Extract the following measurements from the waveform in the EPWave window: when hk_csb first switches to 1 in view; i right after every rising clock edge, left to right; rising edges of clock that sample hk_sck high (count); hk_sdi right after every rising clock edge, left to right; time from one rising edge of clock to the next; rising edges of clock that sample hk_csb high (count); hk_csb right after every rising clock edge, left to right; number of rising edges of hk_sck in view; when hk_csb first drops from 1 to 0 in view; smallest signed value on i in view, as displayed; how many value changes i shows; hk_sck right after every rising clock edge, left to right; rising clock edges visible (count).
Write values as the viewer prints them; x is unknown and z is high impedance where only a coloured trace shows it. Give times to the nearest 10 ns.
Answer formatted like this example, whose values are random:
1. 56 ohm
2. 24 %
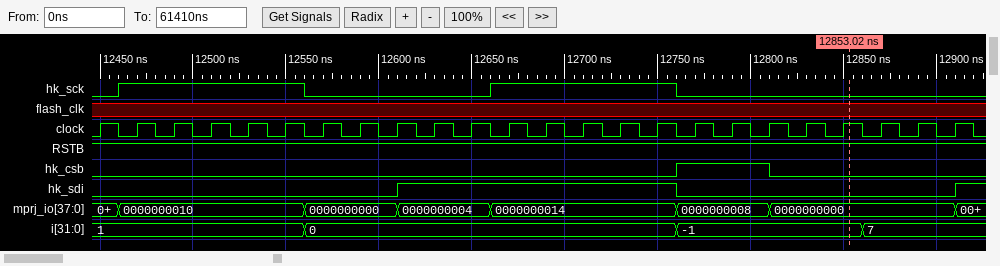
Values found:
1. 12760 ns
2. 1, 1, 1, 1, 1, 1, 0, 0, 0, 0, 0, 0, 0, 0, 0, 0, -1, -1, -1, -1, -1, 7, 7, 7
3. 10
4. 0 0 0 0 0 0 0 0 1 1 1 1 1 1 1 1 0 0 0 0 0 0 0 1
5. 20 ns
6. 3
7. 0 0 0 0 0 0 0 0 0 0 0 0 0 0 0 0 1 1 0 0 0 0 0 0
8. 2
9. 12810 ns
10. -1
11. 3
12. 0 1 1 1 1 1 0 0 0 0 0 1 1 1 1 1 0 0 0 0 0 0 0 0
13. 24
